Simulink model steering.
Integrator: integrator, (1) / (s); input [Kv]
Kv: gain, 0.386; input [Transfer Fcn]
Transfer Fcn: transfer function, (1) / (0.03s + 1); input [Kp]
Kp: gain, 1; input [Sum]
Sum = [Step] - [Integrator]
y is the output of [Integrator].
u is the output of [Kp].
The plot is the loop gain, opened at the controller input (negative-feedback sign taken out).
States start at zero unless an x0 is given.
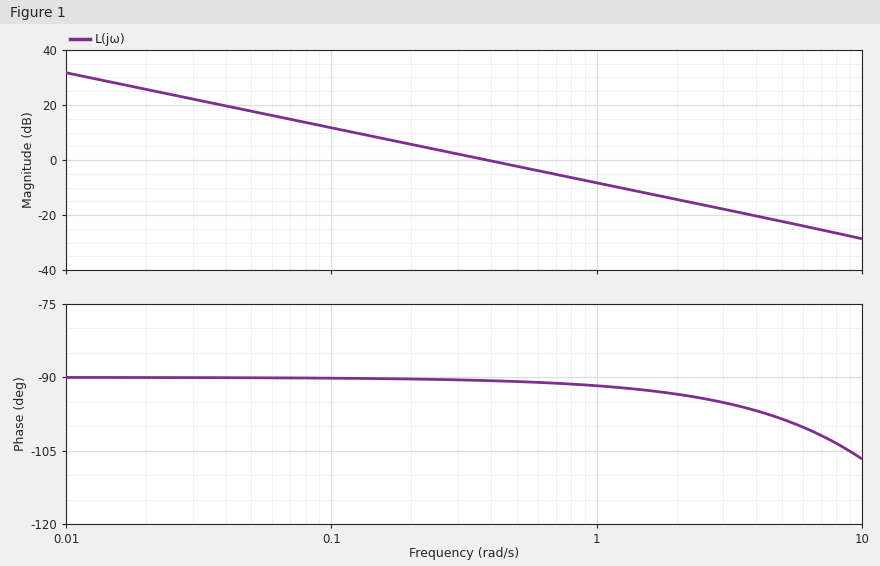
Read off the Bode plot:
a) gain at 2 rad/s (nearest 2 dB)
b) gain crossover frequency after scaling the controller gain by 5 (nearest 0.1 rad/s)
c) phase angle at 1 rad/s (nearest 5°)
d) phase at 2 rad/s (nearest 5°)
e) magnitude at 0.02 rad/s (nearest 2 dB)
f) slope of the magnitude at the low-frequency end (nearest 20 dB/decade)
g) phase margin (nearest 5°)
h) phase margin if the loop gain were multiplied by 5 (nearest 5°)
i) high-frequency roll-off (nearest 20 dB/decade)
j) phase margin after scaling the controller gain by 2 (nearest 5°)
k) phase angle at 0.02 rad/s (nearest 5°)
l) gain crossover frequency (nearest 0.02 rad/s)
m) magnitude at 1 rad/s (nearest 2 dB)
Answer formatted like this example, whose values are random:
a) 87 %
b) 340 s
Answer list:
a) -14 dB
b) 1.9 rad/s
c) -90°
d) -95°
e) 26 dB
f) -20 dB/decade
g) 90°
h) 85°
i) -20 dB/decade
j) 90°
k) -90°
l) 0.38 rad/s
m) -8 dB
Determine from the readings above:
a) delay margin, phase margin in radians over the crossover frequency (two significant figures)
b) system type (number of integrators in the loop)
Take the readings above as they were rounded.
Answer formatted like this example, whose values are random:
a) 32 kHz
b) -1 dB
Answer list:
a) 4.1 s
b) 1
